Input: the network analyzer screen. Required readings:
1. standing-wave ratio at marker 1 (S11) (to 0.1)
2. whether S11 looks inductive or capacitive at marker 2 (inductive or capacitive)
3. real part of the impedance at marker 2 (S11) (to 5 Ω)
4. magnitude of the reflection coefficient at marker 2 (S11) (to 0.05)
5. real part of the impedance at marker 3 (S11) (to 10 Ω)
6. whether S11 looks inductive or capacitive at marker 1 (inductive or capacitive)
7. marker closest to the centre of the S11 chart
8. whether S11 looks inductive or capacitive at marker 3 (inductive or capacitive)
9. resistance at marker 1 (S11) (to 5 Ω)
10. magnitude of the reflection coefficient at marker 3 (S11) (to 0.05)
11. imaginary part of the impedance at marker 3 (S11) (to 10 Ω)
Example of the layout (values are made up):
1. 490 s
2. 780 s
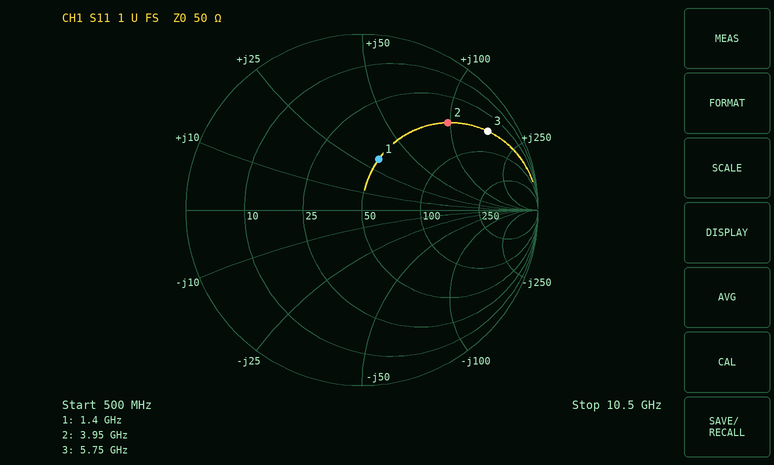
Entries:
1. 1.9
2. inductive
3. 50 Ω
4. 0.70
5. 50 Ω
6. inductive
7. marker 1
8. inductive
9. 50 Ω
10. 0.85
11. +160 Ω
